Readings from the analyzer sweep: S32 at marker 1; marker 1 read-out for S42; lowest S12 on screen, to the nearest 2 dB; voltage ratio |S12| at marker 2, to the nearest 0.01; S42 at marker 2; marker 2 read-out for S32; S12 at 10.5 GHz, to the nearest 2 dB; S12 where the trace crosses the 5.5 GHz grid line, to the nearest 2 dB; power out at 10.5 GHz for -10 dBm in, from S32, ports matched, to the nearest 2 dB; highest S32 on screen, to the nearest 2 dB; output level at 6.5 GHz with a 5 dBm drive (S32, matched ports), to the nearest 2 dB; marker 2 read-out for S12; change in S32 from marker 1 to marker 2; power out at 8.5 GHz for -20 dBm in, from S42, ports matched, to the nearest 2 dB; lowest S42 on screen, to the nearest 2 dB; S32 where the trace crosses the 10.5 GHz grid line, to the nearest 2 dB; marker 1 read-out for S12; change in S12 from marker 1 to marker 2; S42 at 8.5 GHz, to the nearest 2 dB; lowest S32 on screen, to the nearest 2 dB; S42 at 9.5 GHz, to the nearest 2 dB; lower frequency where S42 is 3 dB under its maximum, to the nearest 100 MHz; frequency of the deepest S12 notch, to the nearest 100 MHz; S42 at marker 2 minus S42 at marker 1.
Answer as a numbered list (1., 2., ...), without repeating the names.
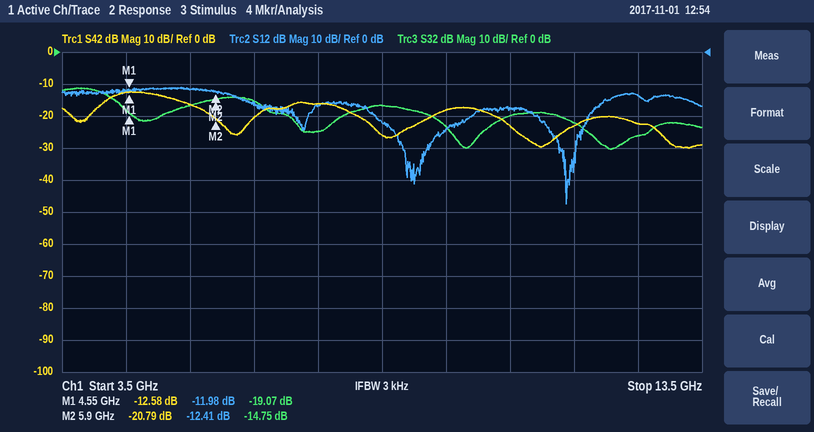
1. -19.07 dB
2. -12.58 dB
3. -48 dB
4. 0.24
5. -20.79 dB
6. -14.75 dB
7. -18 dB
8. -12 dB
9. -30 dBm
10. -12 dB
11. -10 dBm
12. -12.41 dB
13. 4.32 dB
14. -46 dBm
15. -30 dB
16. -20 dB
17. -11.98 dB
18. -0.43 dB
19. -26 dB
20. -30 dB
21. -18 dB
22. 4.2 GHz
23. 11.4 GHz
24. -8.21 dB
